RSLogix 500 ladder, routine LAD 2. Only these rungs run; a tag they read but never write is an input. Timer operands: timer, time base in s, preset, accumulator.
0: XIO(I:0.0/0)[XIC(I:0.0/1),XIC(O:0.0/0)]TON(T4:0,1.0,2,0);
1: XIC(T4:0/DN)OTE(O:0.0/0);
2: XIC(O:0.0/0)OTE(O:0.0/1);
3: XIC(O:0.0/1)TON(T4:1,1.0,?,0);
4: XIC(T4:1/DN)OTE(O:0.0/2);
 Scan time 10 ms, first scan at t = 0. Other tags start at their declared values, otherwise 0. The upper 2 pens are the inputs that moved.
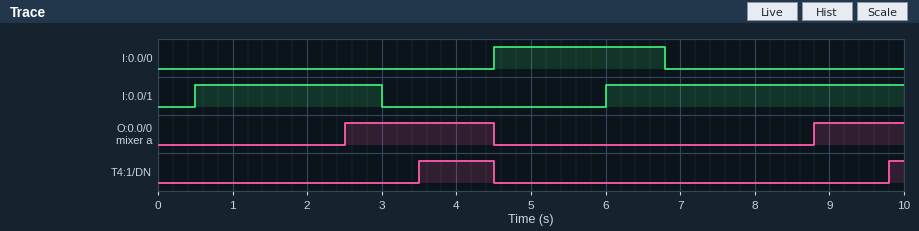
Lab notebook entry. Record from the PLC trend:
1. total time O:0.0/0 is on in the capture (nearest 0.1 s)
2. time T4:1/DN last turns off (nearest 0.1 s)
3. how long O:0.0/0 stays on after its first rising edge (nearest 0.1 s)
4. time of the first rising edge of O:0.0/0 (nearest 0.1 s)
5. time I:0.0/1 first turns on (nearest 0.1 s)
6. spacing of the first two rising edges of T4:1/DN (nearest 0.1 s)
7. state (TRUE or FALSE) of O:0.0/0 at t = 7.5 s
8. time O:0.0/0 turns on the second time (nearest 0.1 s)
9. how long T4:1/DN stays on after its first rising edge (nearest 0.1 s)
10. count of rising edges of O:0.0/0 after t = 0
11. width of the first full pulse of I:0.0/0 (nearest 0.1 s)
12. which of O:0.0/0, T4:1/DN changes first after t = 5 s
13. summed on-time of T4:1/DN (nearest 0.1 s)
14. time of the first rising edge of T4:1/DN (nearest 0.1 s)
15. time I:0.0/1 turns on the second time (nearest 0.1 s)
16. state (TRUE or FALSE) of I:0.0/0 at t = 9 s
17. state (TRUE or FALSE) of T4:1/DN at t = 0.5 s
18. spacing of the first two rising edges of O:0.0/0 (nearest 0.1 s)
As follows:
3.2 s
4.5 s
2.0 s
2.5 s
0.5 s
6.3 s
FALSE
8.8 s
1.0 s
2
2.3 s
O:0.0/0
1.2 s
3.5 s
6.0 s
FALSE
FALSE
6.3 s
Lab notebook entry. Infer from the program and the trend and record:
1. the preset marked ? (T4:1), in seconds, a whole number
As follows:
1 s
